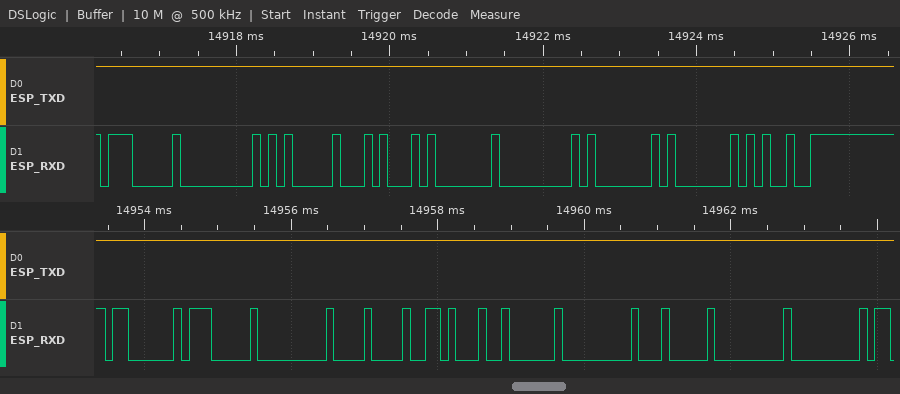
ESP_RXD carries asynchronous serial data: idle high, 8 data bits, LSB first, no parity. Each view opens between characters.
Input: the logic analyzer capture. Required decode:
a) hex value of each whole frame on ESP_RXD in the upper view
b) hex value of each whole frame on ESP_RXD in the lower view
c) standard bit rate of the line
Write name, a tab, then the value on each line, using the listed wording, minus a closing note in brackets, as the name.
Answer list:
hex value of each whole frame on ESP_RXD in the upper view	07, 00, 05, 14, 01, 00, 01, 01, 25
hex value of each whole frame on ESP_RXD in the lower view	03, 07, 00, 08, 16, 02, 00, 04, 00, 00
standard bit rate of the line	9600 baud
